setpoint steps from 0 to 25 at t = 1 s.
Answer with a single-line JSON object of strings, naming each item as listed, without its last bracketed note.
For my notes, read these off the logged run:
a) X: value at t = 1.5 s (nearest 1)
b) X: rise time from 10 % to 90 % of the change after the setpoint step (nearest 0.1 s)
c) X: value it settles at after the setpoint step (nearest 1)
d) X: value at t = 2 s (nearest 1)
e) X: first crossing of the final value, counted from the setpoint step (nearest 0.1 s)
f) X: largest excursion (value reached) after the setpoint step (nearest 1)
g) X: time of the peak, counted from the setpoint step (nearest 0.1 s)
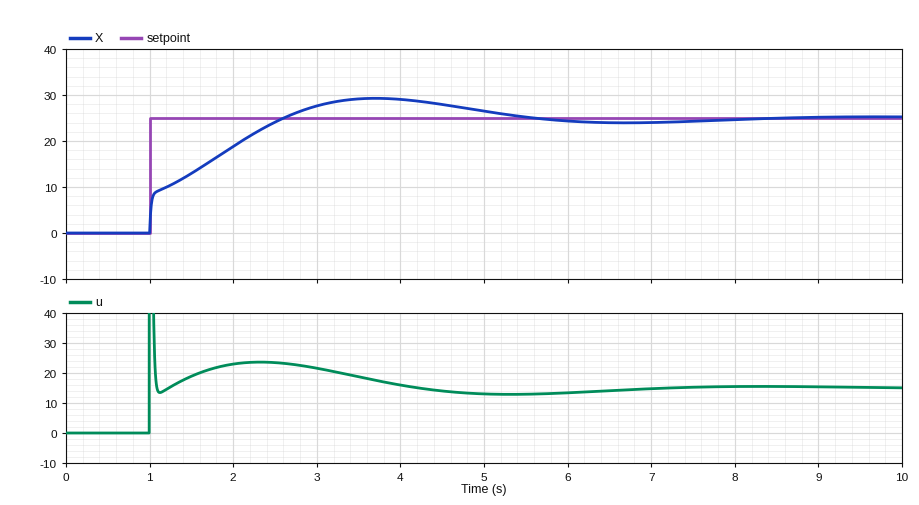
{"X: value at t = 1.5 s": "13", "X: rise time from 10 % to 90 % of the change after the setpoint step": "1.3 s", "X: value it settles at after the setpoint step": "25", "X: value at t = 2 s": "19", "X: first crossing of the final value, counted from the setpoint step": "1.6 s", "X: largest excursion (value reached) after the setpoint step": "29", "X: time of the peak, counted from the setpoint step": "2.7 s"}
